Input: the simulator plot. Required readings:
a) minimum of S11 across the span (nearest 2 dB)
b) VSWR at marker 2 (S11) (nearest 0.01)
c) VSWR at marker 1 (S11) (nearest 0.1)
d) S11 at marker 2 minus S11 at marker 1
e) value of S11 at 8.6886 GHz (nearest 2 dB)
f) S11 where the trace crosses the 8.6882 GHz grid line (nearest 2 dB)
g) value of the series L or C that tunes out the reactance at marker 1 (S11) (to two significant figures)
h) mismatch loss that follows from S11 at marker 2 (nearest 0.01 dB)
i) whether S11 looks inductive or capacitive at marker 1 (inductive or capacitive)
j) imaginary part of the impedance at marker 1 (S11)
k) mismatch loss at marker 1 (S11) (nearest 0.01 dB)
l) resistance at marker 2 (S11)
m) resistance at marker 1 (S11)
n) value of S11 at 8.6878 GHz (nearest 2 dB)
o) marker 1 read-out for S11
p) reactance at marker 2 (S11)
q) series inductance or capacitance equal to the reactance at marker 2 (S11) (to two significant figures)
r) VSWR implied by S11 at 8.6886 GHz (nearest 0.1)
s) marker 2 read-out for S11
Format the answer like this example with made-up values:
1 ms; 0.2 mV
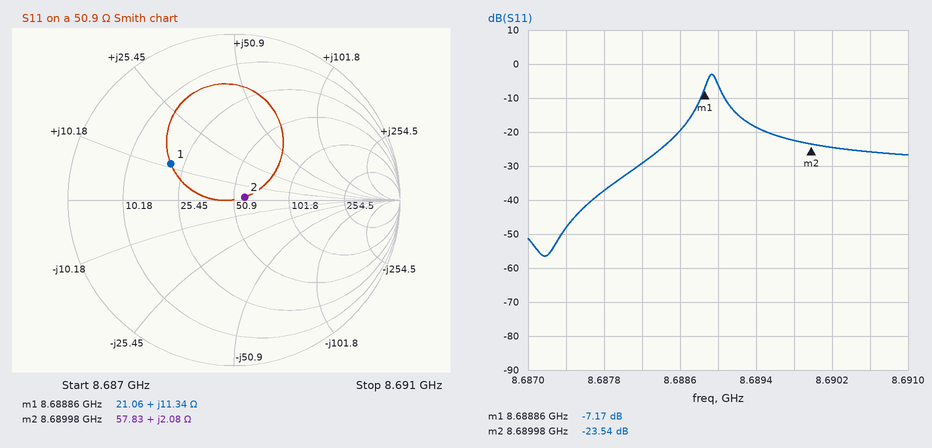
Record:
-56 dB; 1.14; 2.6; -16.37 dB; -20 dB; -30 dB; 1.6 pF; 0.02 dB; inductive; +11.34 Ω; 0.93 dB; 57.83 Ω; 21.06 Ω; -38 dB; -7.17 dB; +2.08 Ω; 38 pH; 1.2; -23.54 dB
